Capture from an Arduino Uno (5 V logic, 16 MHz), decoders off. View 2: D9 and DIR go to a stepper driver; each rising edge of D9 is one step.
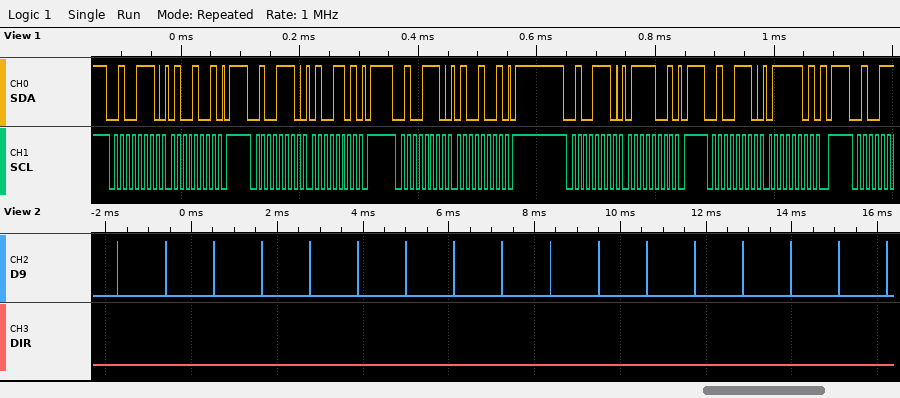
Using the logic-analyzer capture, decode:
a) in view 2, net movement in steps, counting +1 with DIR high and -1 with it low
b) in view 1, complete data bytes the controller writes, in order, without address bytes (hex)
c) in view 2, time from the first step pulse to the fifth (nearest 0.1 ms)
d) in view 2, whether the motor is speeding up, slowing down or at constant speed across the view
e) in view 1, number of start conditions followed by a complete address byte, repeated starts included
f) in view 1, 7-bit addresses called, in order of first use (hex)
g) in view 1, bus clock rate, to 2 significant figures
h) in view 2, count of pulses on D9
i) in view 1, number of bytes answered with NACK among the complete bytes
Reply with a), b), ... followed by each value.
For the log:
a) -17
b) 49 4D 49 79 7D
c) 4.5 ms
d) constant speed
e) 5
f) 0x27
g) 100 kHz
h) 17
i) 0
